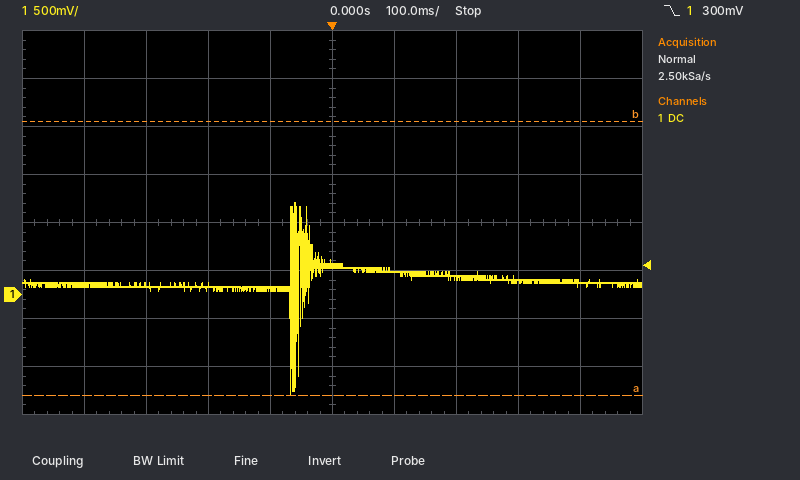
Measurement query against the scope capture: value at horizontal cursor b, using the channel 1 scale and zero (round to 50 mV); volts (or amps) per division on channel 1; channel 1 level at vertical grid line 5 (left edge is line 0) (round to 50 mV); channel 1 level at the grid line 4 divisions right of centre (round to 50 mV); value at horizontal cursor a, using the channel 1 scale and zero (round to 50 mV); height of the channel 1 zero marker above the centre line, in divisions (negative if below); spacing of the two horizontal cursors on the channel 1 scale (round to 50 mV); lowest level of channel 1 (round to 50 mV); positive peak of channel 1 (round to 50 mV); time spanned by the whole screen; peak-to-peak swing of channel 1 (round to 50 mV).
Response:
1.80 V
500 mV
300 mV
100 mV
-1.05 V
-1.5 div
2.85 V
-1.05 V
950 mV
1 s
2.00 V
